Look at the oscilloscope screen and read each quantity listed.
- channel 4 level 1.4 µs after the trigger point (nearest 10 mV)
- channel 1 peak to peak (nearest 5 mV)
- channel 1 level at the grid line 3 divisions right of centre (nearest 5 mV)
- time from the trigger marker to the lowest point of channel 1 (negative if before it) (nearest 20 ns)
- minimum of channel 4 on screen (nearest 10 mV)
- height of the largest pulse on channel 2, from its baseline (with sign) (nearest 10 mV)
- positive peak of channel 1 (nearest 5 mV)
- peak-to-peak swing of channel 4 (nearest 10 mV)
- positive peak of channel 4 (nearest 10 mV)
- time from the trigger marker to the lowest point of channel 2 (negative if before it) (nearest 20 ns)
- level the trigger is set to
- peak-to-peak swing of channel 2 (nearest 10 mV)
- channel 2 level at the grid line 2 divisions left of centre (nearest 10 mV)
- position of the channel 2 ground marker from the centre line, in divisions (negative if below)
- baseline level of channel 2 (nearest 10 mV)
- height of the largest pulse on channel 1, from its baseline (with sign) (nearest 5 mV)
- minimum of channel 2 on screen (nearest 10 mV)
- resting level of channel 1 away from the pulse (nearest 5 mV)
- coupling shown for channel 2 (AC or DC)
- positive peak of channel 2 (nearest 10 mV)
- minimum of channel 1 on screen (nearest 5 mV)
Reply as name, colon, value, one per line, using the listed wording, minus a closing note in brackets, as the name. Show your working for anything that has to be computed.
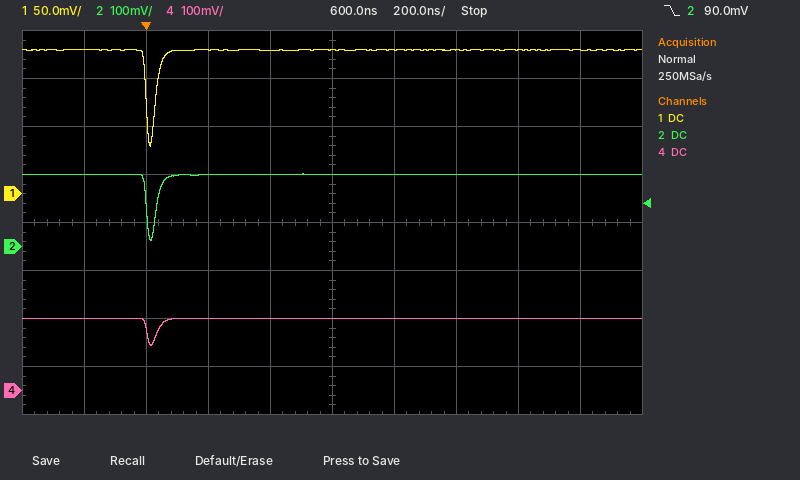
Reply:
channel 4 level 1.4 µs after the trigger point: 150 mV
channel 1 peak to peak: 150 mV − (50 mV) = 100 mV
channel 1 level at the grid line 3 divisions right of centre: 150 mV
time from the trigger marker to the lowest point of channel 1 (negative if before it): +20 ns
minimum of channel 4 on screen: 90 mV
height of the largest pulse on channel 2, from its baseline (with sign): 10 mV − (150 mV) = -140 mV
positive peak of channel 1: 150 mV
peak-to-peak swing of channel 4: 150 mV − (90 mV) = 60 mV
positive peak of channel 4: 150 mV
time from the trigger marker to the lowest point of channel 2 (negative if before it): +20 ns
level the trigger is set to: 90.0 mV
peak-to-peak swing of channel 2: 150 mV − (10 mV) = 140 mV
channel 2 level at the grid line 2 divisions left of centre: 150 mV
position of the channel 2 ground marker from the centre line, in divisions: -0.5 div
baseline level of channel 2: 150 mV
height of the largest pulse on channel 1, from its baseline (with sign): 50 mV − (150 mV) = -100 mV
minimum of channel 2 on screen: 10 mV
resting level of channel 1 away from the pulse: 150 mV
coupling shown for channel 2: DC
positive peak of channel 2: 150 mV
minimum of channel 1 on screen: 50 mV
